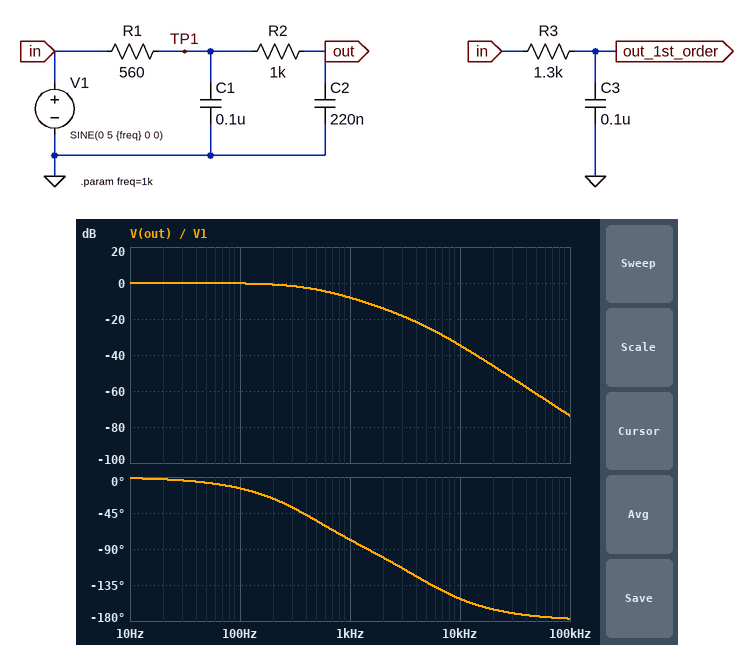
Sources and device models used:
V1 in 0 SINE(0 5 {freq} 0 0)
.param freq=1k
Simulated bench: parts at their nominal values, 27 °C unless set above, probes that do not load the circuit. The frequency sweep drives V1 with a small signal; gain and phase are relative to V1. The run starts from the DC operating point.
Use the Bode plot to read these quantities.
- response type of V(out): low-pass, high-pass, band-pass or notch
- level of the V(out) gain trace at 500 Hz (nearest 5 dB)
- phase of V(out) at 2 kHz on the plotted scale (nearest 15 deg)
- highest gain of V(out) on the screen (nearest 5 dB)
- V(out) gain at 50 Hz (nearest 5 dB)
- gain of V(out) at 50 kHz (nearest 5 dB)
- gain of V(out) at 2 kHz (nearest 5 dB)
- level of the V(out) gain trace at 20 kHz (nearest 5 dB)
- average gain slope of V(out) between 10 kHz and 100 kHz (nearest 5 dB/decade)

low-pass
-5 dB
-105 deg
0 dB
0 dB
-60 dB
-15 dB
-45 dB
-40 dB/decade
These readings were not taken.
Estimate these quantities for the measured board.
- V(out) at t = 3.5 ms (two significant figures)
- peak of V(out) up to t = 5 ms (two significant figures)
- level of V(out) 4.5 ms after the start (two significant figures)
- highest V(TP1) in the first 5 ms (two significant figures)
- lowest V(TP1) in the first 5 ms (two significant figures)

1.9 V
2.5 V
1.9 V
3.7 V
-3.3 V
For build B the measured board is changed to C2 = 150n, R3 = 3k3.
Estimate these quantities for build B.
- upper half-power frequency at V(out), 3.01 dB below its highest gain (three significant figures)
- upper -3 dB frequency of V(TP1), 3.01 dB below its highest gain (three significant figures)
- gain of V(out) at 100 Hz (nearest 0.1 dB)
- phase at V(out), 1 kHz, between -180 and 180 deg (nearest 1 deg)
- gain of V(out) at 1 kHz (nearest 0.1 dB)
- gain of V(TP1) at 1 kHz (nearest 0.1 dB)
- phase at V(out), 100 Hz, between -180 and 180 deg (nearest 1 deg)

609 Hz
1.00 kHz
-0.1 dB
-70 deg
-5.8 dB
-3.0 dB
-10 deg
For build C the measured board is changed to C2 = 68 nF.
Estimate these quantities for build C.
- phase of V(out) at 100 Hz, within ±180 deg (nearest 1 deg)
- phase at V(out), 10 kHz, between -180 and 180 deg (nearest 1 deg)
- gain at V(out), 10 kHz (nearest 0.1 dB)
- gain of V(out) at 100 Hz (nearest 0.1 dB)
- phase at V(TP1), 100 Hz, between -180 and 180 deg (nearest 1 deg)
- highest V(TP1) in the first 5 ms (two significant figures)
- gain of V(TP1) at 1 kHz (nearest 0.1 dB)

-6 deg
-144 deg
-24.8 dB
0 dB
-3 deg
4.2 V
-1.7 dB
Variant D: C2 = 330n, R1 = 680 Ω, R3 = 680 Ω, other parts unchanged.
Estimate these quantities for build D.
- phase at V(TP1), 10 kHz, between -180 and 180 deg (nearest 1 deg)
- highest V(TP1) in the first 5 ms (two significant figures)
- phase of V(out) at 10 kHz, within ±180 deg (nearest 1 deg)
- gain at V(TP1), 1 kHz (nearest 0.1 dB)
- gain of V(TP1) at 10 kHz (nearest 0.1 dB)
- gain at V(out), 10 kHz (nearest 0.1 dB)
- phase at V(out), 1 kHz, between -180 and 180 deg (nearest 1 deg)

-69 deg
3.3 V
-156 deg
-4.6 dB
-13.3 dB
-39.6 dB
-88 deg
